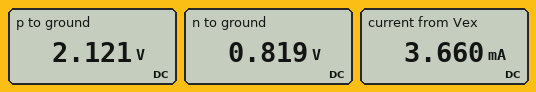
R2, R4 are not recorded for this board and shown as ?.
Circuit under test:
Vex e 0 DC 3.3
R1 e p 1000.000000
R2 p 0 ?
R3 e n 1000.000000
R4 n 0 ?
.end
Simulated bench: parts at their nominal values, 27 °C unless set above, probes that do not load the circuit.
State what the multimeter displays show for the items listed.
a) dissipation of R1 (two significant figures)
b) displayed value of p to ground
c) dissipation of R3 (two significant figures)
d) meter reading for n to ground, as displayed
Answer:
1.4 mW
2.121 V
6.2 mW
0.819 V
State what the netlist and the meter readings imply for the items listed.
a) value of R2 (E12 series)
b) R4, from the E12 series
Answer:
1.8 kΩ
330 Ω
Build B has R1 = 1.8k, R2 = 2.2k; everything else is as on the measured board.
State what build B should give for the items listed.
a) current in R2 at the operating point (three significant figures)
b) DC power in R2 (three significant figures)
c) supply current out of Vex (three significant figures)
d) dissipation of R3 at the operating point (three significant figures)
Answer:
825 µA
1.50 mW
3.31 mA
6.16 mW
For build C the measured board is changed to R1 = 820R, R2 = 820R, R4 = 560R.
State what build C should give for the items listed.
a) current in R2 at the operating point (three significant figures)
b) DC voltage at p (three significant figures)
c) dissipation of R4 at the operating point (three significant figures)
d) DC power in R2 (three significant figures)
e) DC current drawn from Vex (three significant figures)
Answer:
2.01 mA
1.65 V
2.51 mW
3.32 mW
4.13 mA
